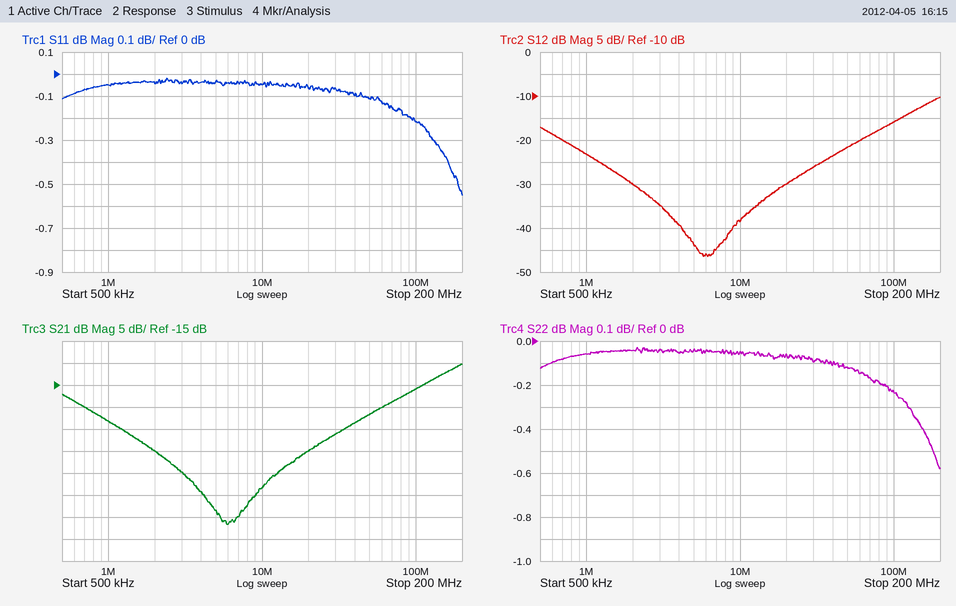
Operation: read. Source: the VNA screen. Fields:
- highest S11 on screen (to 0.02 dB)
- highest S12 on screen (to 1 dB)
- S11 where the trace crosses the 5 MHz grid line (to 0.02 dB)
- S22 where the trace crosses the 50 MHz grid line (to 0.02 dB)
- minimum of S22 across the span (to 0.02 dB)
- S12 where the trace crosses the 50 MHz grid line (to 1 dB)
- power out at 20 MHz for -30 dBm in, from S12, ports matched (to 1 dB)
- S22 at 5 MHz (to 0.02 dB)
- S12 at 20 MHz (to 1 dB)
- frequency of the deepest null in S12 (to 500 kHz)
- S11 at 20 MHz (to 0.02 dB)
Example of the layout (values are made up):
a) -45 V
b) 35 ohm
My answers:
a) -0.02 dB
b) -10 dB
c) -0.04 dB
d) -0.12 dB
e) -0.58 dB
f) -22 dB
g) -60 dBm
h) -0.04 dB
i) -30 dB
j) 6.0 MHz
k) -0.06 dB
